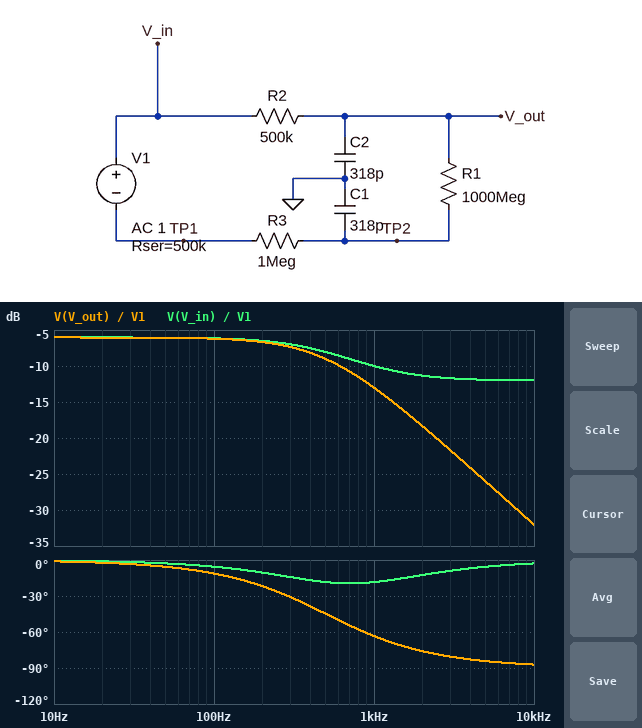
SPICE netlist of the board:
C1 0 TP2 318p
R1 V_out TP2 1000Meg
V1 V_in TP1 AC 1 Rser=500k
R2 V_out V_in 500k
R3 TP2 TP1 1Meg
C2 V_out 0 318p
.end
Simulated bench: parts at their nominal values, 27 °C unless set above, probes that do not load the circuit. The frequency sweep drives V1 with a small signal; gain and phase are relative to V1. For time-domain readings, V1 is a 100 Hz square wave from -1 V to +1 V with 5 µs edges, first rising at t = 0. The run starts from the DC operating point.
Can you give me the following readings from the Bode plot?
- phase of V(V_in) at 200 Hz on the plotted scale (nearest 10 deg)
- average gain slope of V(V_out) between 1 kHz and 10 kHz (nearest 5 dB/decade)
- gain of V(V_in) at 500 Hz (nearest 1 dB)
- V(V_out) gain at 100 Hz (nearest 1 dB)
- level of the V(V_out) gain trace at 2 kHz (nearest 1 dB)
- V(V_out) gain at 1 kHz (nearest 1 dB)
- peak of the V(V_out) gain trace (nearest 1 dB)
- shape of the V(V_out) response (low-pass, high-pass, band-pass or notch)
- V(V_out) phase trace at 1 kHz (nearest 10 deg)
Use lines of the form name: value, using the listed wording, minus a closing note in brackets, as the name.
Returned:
phase of V(V_in) at 200 Hz on the plotted scale: -10 deg
average gain slope of V(V_out) between 1 kHz and 10 kHz: -20 dB/decade
gain of V(V_in) at 500 Hz: -8 dB
V(V_out) gain at 100 Hz: -6 dB
level of the V(V_out) gain trace at 2 kHz: -18 dB
V(V_out) gain at 1 kHz: -13 dB
peak of the V(V_out) gain trace: -6 dB
shape of the V(V_out) response: low-pass
V(V_out) phase trace at 1 kHz: -60 deg
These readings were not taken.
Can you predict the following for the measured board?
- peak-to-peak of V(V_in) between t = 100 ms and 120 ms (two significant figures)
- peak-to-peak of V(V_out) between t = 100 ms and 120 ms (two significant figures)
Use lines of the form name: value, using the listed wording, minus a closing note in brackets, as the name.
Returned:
peak-to-peak of V(V_in) between t = 100 ms and 120 ms: 1.0 V
peak-to-peak of V(V_out) between t = 100 ms and 120 ms: 1.0 V
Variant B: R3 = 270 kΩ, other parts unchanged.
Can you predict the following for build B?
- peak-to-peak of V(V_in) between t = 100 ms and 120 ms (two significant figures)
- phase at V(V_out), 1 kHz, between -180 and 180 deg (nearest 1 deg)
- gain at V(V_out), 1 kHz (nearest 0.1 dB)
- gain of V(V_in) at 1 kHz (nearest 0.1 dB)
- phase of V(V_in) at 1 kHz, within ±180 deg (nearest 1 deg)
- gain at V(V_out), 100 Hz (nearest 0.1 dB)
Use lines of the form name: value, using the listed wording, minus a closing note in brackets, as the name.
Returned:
peak-to-peak of V(V_in) between t = 100 ms and 120 ms: 1.0 V
phase at V(V_out), 1 kHz, between -180 and 180 deg: -52 deg
gain at V(V_out), 1 kHz: -10.2 dB
gain of V(V_in) at 1 kHz: -7.2 dB
phase of V(V_in) at 1 kHz, within ±180 deg: -7 deg
gain at V(V_out), 100 Hz: -6.1 dB
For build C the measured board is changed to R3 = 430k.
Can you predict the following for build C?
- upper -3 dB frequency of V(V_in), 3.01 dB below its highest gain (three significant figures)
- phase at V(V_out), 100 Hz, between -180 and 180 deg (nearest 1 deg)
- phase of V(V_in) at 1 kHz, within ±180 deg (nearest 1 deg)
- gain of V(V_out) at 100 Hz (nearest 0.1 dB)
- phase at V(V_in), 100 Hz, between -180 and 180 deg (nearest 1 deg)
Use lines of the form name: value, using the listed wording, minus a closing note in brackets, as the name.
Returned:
upper -3 dB frequency of V(V_in), 3.01 dB below its highest gain: 4.82 kHz
phase at V(V_out), 100 Hz, between -180 and 180 deg: -8 deg
phase of V(V_in) at 1 kHz, within ±180 deg: -10 deg
gain of V(V_out) at 100 Hz: -6.1 dB
phase at V(V_in), 100 Hz, between -180 and 180 deg: -2 deg
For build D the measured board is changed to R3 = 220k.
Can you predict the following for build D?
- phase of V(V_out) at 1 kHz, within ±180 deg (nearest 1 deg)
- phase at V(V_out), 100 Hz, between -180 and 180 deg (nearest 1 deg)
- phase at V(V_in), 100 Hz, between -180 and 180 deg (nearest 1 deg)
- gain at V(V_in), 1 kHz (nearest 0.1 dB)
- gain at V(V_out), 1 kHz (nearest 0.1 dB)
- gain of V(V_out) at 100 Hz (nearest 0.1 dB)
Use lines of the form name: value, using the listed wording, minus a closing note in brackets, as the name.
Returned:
phase of V(V_out) at 1 kHz, within ±180 deg: -51 deg
phase at V(V_out), 100 Hz, between -180 and 180 deg: -7 deg
phase at V(V_in), 100 Hz, between -180 and 180 deg: -1 deg
gain at V(V_in), 1 kHz: -7.0 dB
gain at V(V_out), 1 kHz: -10.0 dB
gain of V(V_out) at 100 Hz: -6.1 dB
